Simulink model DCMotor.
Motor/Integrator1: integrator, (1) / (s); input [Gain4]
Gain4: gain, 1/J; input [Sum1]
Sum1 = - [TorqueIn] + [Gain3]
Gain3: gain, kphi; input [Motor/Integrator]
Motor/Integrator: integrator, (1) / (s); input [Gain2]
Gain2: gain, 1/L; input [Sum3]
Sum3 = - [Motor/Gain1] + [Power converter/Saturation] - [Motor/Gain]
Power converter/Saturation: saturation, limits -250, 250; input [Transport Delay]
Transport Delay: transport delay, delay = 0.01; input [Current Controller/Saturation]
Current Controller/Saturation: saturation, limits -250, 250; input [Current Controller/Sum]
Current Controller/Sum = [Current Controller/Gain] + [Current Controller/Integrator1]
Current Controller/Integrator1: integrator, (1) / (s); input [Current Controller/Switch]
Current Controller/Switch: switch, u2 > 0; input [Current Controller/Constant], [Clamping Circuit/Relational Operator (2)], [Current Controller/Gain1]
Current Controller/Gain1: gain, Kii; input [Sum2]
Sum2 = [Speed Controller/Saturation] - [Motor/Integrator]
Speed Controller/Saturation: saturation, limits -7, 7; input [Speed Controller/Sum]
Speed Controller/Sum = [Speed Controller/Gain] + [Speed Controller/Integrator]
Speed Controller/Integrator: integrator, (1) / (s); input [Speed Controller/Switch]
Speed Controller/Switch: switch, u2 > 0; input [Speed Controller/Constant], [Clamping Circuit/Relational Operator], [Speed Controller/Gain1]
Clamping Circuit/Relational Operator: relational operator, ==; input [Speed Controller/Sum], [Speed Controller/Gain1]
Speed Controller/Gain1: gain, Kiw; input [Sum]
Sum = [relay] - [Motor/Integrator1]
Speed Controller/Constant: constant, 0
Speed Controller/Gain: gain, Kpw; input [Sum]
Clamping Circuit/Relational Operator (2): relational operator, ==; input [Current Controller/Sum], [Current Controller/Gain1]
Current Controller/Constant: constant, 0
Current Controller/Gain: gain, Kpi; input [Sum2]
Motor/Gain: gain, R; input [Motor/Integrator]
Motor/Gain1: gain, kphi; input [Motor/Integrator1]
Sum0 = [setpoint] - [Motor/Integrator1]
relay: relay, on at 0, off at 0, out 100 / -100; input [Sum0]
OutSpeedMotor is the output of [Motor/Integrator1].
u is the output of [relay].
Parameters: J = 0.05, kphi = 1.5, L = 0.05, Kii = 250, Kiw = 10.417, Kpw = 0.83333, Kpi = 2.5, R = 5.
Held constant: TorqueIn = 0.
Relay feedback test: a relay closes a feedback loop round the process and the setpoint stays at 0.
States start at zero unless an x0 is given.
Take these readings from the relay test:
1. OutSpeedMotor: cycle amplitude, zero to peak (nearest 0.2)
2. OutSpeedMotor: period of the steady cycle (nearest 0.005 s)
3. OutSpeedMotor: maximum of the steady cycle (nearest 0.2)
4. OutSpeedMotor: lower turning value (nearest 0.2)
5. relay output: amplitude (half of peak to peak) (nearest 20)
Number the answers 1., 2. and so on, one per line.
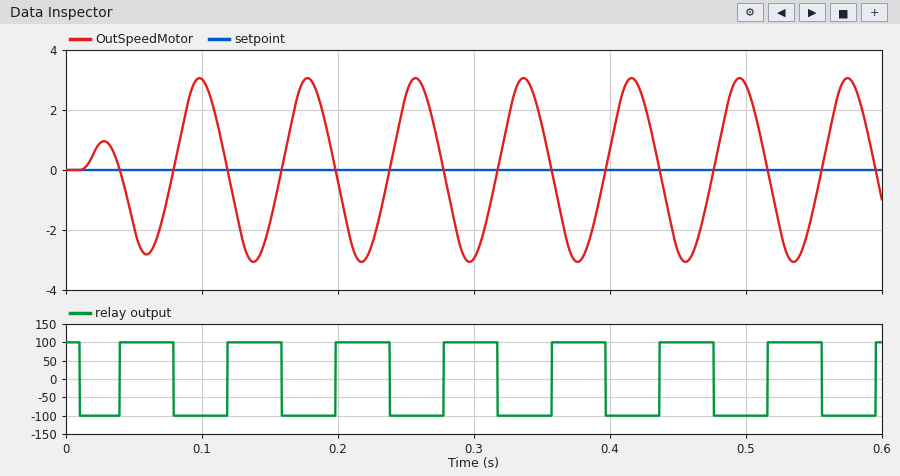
1. 3.0
2. 0.080 s
3. 3.0
4. -3.0
5. 100
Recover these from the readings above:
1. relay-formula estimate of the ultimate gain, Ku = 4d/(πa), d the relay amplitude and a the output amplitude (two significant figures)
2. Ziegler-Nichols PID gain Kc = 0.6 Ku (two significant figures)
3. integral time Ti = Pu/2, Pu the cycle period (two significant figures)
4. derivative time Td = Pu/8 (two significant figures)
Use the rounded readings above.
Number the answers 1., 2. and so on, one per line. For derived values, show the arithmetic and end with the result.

1. 4 × 100 / (π × 3) = 42
2. 0.6 × 42 = 25
3. 0.08 / 2 = 0.040 s
4. 0.08 / 8 = 0.010 s
